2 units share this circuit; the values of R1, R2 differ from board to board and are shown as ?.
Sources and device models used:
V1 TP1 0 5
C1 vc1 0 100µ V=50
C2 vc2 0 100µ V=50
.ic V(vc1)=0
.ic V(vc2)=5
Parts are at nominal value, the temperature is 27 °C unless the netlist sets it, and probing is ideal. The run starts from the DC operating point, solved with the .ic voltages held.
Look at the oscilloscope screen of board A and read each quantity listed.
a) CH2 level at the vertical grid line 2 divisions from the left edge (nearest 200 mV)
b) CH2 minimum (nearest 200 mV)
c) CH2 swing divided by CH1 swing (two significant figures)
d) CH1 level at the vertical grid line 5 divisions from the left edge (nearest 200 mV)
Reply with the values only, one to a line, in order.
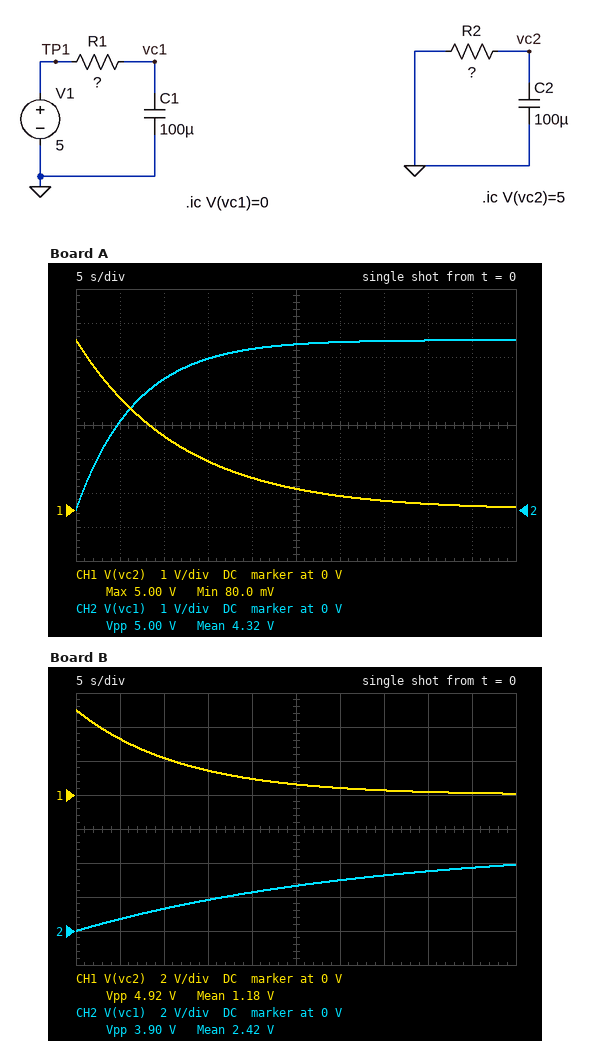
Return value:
3.8 V
0 V
1.0
600 mV
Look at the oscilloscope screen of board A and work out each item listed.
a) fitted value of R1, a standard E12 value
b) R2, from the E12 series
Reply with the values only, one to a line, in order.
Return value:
68 kΩ
120 kΩ
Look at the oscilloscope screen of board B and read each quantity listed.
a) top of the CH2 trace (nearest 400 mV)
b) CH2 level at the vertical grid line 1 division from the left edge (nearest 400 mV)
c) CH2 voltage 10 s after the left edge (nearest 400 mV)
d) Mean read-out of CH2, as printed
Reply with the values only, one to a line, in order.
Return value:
4.0 V
800 mV
1.2 V
2.42 V
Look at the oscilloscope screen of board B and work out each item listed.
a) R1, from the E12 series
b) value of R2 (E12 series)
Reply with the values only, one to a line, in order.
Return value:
330 kΩ
120 kΩ
